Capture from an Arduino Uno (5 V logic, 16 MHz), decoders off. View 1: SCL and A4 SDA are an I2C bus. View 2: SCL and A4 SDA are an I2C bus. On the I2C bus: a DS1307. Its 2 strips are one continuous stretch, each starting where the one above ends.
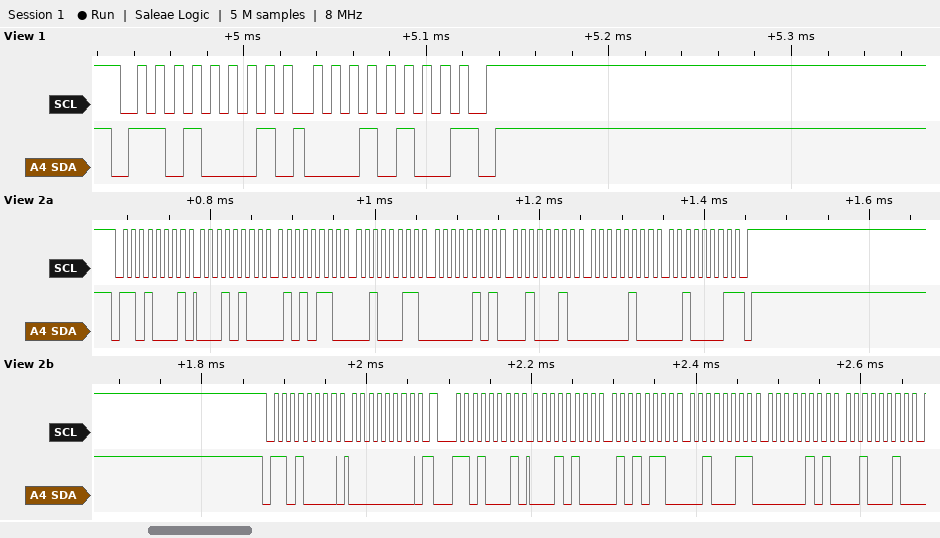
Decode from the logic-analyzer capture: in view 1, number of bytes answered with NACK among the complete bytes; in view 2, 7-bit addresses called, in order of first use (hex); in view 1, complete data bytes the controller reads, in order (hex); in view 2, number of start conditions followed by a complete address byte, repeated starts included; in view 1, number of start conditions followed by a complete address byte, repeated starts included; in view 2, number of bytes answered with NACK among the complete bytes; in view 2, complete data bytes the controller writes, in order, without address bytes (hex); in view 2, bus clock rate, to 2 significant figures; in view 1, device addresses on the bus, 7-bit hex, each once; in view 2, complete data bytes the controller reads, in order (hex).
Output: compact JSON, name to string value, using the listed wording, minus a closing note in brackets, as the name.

{"in view 1, number of bytes answered with NACK among the complete bytes": "1", "in view 2, 7-bit addresses called, in order of first use": "0x68", "in view 1, complete data bytes the controller reads, in order": "14", "in view 2, number of start conditions followed by a complete address byte, repeated starts included": "3", "in view 1, number of start conditions followed by a complete address byte, repeated starts included": "1", "in view 2, number of bytes answered with NACK among the complete bytes": "1", "in view 2, complete data bytes the controller writes, in order, without address bytes": "00", "in view 2, bus clock rate, to 2 significant figures": "100 kHz", "in view 1, device addresses on the bus, 7-bit hex, each once": "0x68", "in view 2, complete data bytes the controller reads, in order": "14 56 23 05 22 04 21 14 56 23 05 22"}
